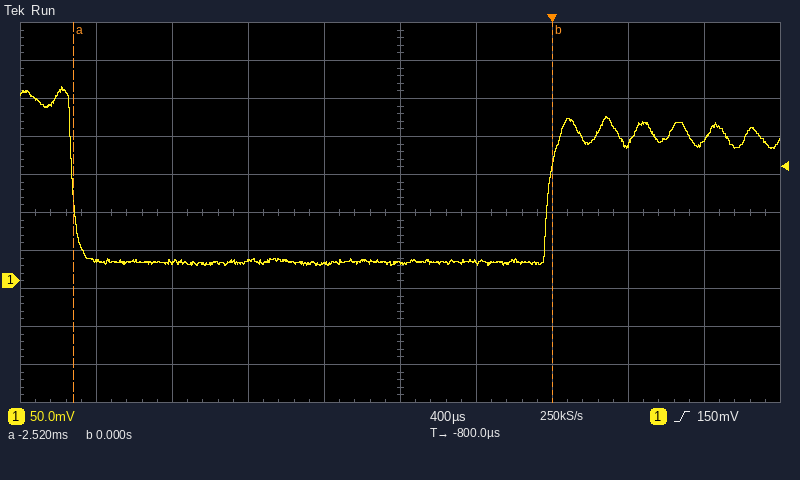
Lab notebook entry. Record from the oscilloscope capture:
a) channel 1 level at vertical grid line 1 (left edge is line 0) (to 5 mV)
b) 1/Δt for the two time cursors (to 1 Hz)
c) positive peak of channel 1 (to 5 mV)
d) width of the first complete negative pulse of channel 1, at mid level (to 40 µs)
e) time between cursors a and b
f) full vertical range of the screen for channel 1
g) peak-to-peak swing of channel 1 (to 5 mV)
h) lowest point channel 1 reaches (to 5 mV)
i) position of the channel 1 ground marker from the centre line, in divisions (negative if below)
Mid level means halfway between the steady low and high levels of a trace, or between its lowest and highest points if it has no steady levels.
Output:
25 mV
397 Hz
255 mV
2.52 ms
2.52 ms
500 mV
235 mV
20 mV
-1.8 div
